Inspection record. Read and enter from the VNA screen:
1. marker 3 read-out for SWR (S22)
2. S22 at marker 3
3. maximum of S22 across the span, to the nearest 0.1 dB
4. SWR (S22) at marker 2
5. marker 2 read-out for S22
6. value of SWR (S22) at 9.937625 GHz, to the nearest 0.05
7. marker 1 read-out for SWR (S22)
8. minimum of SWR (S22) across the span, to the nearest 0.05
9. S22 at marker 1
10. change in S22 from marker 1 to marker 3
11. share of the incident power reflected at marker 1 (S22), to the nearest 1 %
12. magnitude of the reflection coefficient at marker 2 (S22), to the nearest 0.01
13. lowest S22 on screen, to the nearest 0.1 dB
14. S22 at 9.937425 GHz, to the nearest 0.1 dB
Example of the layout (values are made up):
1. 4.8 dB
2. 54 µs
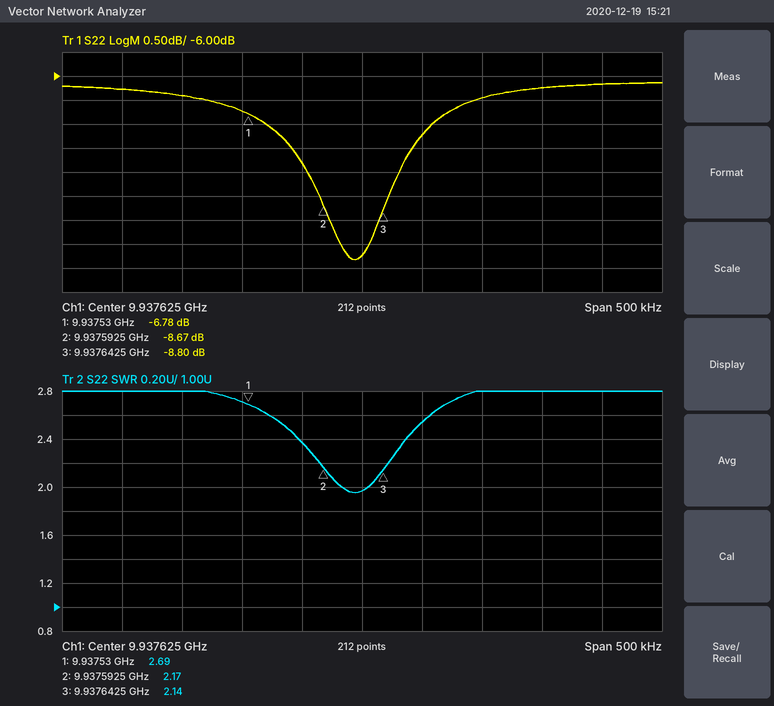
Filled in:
1. 2.14
2. -8.80 dB
3. -6.1 dB
4. 2.17
5. -8.67 dB
6. 1.95
7. 2.69
8. 1.95
9. -6.78 dB
10. -2.02 dB
11. 21 %
12. 0.37
13. -9.8 dB
14. -6.3 dB
